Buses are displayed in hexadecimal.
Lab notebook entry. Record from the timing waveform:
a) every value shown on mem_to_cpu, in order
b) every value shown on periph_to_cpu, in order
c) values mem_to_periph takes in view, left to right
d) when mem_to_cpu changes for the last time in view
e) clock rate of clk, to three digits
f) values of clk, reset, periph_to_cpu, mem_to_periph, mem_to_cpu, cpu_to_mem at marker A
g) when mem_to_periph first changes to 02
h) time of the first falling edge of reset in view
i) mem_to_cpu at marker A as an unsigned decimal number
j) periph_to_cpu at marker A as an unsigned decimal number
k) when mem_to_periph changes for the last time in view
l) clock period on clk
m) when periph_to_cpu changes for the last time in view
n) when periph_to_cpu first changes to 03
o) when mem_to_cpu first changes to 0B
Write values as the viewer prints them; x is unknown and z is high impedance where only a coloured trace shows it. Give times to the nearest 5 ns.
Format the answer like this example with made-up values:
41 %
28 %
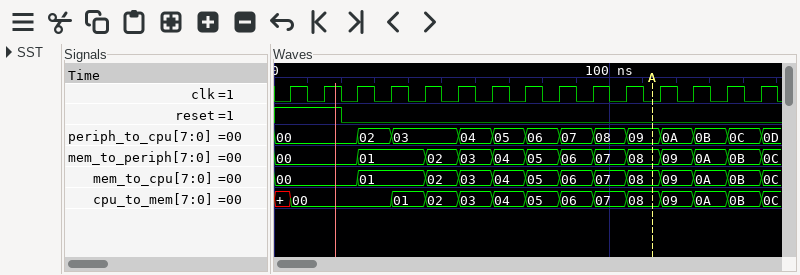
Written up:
00, 01, 02, 03, 04, 05, 06, 07, 08, 09, 0A, 0B, 0C
00, 02, 03, 04, 05, 06, 07, 08, 09, 0A, 0B, 0C, 0D
00, 01, 02, 03, 04, 05, 06, 07, 08, 09, 0A, 0B, 0C
145 ns
100 MHz
clk=0, reset=0, periph_to_cpu=09, mem_to_periph=08, mem_to_cpu=08, cpu_to_mem=08
45 ns
20 ns
8
9
145 ns
10 ns
145 ns
35 ns
135 ns
